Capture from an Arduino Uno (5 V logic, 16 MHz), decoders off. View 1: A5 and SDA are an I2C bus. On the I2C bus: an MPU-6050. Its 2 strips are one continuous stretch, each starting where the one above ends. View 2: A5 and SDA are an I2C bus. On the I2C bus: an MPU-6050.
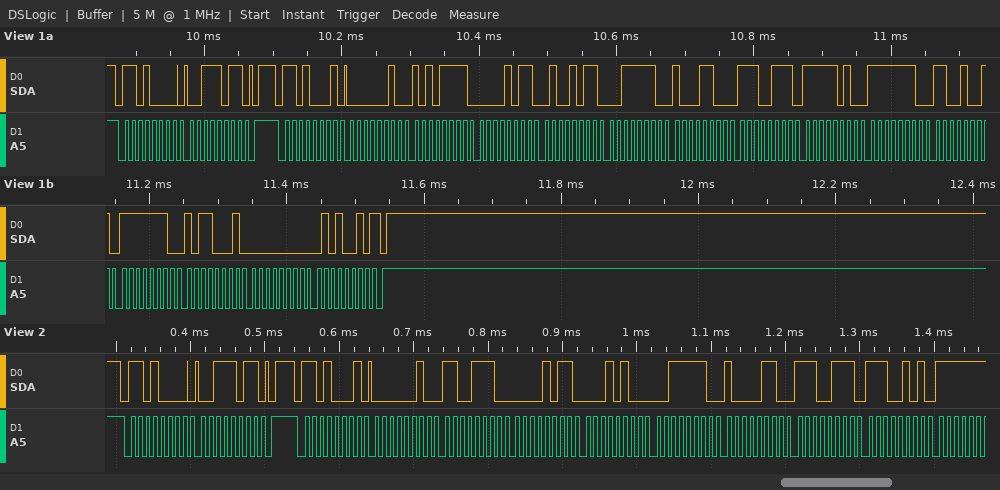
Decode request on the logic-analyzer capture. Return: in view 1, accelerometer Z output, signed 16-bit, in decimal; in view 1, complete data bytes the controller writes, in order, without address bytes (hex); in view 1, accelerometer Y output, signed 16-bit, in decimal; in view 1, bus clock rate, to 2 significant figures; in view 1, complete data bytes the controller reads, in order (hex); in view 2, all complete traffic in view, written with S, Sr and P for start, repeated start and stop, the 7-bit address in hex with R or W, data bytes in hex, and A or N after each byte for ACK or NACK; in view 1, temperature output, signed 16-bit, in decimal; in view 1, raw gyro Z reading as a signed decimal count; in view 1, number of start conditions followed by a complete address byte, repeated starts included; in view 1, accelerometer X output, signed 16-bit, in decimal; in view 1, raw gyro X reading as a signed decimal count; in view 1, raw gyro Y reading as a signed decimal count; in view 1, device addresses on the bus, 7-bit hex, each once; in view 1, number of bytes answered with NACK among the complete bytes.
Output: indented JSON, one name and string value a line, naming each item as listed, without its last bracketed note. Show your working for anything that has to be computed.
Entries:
{
  "in view 1, accelerometer Z output, signed 16-bit, in decimal": "0x3E8C = 16012",
  "in view 1, complete data bytes the controller writes, in order, without address bytes": "3B",
  "in view 1, accelerometer Y output, signed 16-bit, in decimal": "0x0B4B = 2891",
  "in view 1, bus clock rate, to 2 significant figures": "100 kHz",
  "in view 1, complete data bytes the controller reads, in order": "02 AF 0B 4B 3E 8C E7 FA FE C9 FE B1 00 52",
  "in view 2, all complete traffic in view, written with S, Sr and P for start, repeated start and stop, the 7-bit address in hex with R or W, data bytes in hex, and A or N after each byte for ACK or NACK": "S 68W A 3B A P S 68R A 02 A CE A 0B A 14 A 3E A 86 A E7 A E5 A",
  "in view 1, temperature output, signed 16-bit, in decimal": "0xE7FA = -6150",
  "in view 1, raw gyro Z reading as a signed decimal count": "0x0052 = 82",
  "in view 1, number of start conditions followed by a complete address byte, repeated starts included": "2",
  "in view 1, accelerometer X output, signed 16-bit, in decimal": "0x02AF = 687",
  "in view 1, raw gyro X reading as a signed decimal count": "0xFEC9 = -311",
  "in view 1, raw gyro Y reading as a signed decimal count": "0xFEB1 = -335",
  "in view 1, device addresses on the bus, 7-bit hex, each once": "0x68",
  "in view 1, number of bytes answered with NACK among the complete bytes": "1"
}
